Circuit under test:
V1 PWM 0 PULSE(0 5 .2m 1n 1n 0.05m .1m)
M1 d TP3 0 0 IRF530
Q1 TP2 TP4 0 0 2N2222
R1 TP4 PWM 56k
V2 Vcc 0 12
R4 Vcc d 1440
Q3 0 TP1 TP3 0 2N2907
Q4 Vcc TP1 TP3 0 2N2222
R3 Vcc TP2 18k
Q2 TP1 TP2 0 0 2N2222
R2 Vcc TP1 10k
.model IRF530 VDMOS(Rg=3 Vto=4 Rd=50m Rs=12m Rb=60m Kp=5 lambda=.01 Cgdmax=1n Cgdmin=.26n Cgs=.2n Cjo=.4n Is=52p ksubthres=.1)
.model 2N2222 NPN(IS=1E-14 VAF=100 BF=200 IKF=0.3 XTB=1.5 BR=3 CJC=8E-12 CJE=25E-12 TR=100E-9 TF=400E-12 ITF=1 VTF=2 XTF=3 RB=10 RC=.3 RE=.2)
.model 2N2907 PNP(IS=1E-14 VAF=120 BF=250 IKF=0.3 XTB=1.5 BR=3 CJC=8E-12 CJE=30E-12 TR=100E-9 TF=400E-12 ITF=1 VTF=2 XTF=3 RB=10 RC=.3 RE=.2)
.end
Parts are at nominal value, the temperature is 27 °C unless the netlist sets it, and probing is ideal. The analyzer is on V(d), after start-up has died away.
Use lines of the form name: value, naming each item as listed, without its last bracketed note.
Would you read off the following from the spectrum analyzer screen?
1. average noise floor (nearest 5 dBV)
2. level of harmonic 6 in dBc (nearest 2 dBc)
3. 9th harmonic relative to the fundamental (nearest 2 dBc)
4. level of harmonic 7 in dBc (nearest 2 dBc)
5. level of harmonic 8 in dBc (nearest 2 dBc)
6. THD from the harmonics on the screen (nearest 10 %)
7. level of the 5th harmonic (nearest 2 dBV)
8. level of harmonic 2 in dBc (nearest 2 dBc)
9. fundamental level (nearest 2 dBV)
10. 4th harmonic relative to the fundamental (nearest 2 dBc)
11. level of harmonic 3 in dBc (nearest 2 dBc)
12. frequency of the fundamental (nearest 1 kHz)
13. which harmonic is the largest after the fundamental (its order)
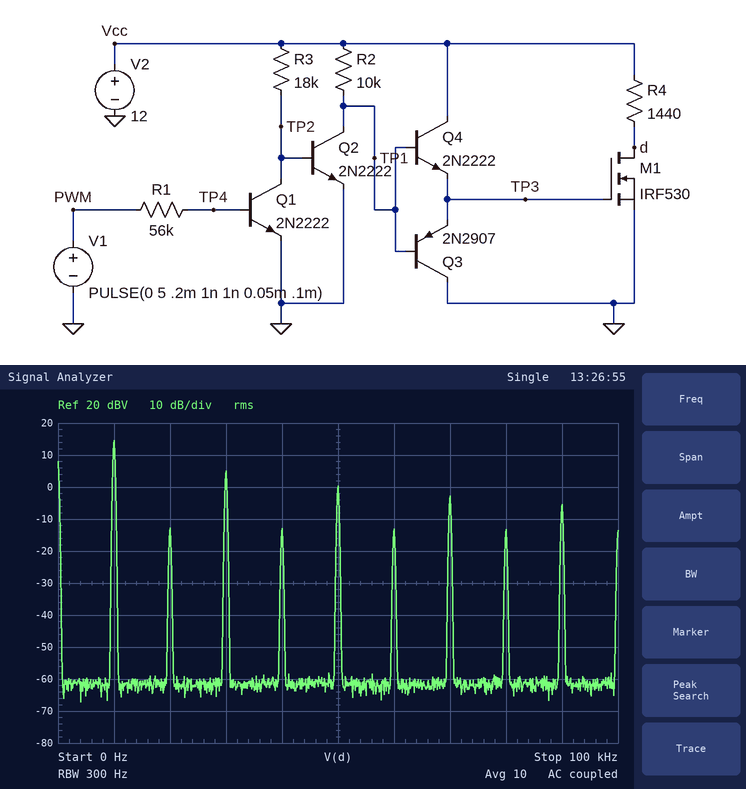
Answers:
average noise floor: -60 dBV
level of harmonic 6 in dBc: -28 dBc
9th harmonic relative to the fundamental: -20 dBc
level of harmonic 7 in dBc: -18 dBc
level of harmonic 8 in dBc: -28 dBc
THD from the harmonics on the screen: 40 %
level of the 5th harmonic: 0 dBV
level of harmonic 2 in dBc: -28 dBc
fundamental level: 14 dBV
4th harmonic relative to the fundamental: -28 dBc
level of harmonic 3 in dBc: -10 dBc
frequency of the fundamental: 10 kHz
which harmonic is the largest after the fundamental: 3
